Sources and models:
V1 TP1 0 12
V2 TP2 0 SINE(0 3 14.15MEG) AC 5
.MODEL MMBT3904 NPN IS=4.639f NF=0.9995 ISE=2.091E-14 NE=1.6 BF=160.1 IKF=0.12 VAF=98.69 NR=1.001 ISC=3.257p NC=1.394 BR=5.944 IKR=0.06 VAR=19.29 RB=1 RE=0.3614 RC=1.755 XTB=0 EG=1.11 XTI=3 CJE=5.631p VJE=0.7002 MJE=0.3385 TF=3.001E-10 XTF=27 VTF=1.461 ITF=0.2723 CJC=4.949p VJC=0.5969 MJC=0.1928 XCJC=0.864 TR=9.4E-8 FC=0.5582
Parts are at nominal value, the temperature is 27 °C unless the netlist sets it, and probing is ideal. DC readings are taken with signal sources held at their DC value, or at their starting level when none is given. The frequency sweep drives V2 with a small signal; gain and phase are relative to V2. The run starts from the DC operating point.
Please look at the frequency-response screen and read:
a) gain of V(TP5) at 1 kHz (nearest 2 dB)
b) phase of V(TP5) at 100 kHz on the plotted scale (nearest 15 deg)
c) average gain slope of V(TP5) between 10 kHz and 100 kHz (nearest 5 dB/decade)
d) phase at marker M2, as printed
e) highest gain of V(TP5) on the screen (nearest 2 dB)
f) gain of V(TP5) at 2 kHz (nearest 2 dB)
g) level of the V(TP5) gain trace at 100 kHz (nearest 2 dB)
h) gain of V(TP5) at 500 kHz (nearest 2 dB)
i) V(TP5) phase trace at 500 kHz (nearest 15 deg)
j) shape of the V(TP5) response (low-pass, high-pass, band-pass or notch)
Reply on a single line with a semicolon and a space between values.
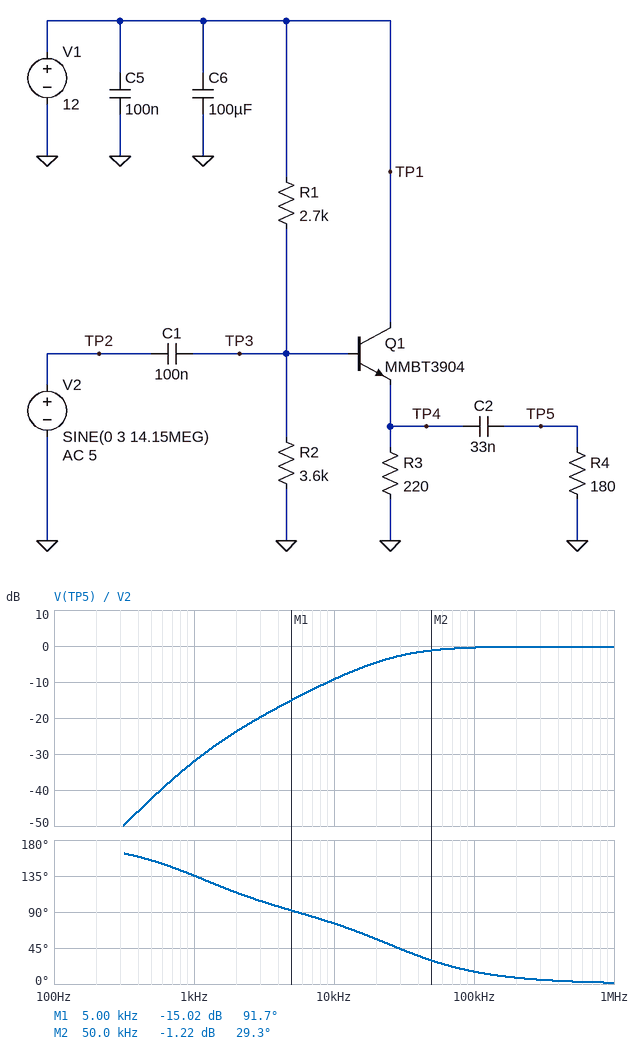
-32 dB; 15 deg; 10 dB/decade; 29.3 deg; 0 dB; -24 dB; 0 dB; 0 dB; 0 deg; high-pass
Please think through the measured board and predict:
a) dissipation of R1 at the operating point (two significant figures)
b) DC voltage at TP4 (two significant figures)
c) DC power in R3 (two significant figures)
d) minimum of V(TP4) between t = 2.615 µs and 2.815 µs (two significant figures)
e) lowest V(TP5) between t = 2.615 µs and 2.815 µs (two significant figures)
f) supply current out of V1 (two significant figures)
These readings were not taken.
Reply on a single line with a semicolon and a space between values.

11 mW; 5.8 V; 150 mW; 3.1 V; -2.7 V; 28 mA
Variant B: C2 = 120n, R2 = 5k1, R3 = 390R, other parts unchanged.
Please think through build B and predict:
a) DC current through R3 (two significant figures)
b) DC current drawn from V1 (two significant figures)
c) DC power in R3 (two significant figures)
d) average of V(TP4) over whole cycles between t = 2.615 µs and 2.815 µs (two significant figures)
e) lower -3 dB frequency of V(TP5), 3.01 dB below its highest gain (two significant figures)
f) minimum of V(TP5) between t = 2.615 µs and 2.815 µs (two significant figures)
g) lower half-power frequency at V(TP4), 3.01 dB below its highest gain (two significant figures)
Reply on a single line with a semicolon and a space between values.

18 mA; 19 mA; 120 mW; 7.0 V; 7.5 kHz; -2.3 V; 930 Hz
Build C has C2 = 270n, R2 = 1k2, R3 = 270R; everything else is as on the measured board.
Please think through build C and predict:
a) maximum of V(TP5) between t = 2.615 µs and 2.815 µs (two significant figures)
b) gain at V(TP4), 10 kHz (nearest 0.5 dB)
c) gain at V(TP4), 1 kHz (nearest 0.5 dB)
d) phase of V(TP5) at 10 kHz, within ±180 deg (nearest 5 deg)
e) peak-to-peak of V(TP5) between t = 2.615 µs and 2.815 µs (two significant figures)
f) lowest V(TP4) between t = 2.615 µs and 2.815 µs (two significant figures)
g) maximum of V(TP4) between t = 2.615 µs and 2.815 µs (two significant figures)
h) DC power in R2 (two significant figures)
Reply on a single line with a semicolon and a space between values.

2.9 V; -0.5 dB; -7.0 dB; 30 deg; 4.3 V; 1.6 V; 5.8 V; 11 mW
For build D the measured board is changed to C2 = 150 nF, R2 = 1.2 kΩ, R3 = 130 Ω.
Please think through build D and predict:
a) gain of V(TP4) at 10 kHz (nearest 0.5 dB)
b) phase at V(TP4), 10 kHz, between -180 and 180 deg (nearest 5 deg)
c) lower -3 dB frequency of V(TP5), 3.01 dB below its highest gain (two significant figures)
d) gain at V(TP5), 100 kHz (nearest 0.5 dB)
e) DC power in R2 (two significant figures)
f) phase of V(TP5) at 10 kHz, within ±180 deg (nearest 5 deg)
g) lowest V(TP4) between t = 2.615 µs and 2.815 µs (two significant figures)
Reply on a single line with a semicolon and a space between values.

-0.5 dB; 10 deg; 6.5 kHz; 0 dB; 11 mW; 40 deg; 1.1 V
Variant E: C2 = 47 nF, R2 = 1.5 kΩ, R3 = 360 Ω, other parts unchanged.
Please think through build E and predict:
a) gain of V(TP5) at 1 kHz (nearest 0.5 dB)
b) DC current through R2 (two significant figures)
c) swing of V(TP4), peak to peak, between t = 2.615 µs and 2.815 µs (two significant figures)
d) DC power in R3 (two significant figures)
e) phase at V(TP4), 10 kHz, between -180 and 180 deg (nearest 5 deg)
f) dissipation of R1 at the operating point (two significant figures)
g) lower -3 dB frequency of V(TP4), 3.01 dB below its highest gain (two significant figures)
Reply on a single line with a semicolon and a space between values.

-31.5 dB; 2.8 mA; 4.2 V; 34 mW; 10 deg; 22 mW; 1.6 kHz
